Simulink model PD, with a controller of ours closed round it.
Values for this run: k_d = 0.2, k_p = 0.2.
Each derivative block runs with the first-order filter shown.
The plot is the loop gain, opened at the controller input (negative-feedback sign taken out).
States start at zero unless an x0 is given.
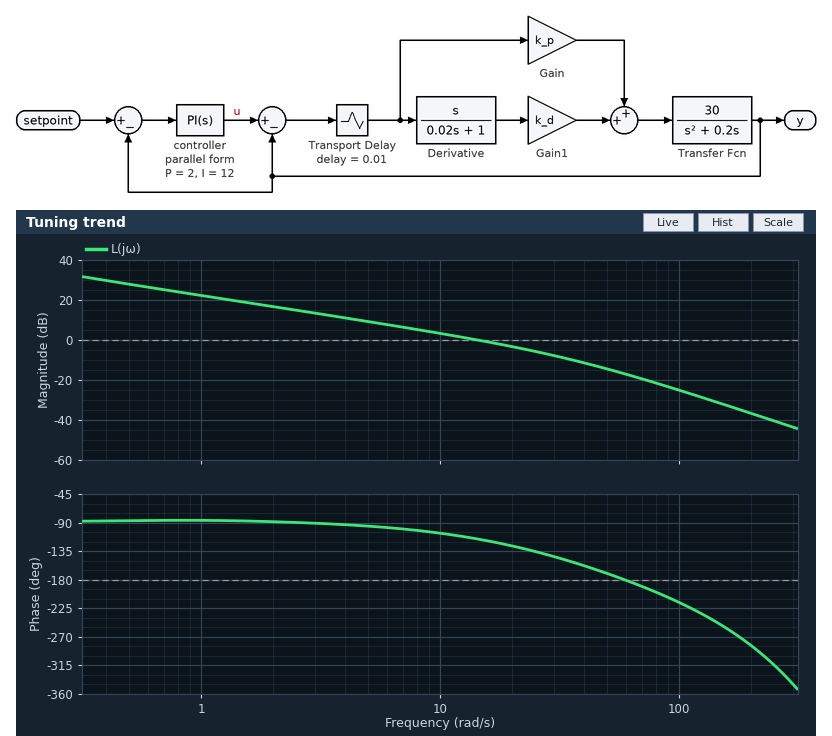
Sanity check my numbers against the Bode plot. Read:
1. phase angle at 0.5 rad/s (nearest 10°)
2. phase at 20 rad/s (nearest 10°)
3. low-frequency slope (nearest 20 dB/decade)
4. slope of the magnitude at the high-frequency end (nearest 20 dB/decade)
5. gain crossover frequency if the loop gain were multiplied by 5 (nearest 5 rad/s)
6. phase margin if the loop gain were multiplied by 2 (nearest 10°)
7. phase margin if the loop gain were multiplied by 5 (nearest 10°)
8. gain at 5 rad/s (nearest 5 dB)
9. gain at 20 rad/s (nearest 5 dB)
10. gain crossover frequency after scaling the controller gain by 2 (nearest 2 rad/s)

-90°
-130°
-20 dB/decade
-40 dB/decade
50 rad/s
40°
10°
10 dB
-5 dB
26 rad/s
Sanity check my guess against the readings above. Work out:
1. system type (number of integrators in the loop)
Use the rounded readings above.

1
